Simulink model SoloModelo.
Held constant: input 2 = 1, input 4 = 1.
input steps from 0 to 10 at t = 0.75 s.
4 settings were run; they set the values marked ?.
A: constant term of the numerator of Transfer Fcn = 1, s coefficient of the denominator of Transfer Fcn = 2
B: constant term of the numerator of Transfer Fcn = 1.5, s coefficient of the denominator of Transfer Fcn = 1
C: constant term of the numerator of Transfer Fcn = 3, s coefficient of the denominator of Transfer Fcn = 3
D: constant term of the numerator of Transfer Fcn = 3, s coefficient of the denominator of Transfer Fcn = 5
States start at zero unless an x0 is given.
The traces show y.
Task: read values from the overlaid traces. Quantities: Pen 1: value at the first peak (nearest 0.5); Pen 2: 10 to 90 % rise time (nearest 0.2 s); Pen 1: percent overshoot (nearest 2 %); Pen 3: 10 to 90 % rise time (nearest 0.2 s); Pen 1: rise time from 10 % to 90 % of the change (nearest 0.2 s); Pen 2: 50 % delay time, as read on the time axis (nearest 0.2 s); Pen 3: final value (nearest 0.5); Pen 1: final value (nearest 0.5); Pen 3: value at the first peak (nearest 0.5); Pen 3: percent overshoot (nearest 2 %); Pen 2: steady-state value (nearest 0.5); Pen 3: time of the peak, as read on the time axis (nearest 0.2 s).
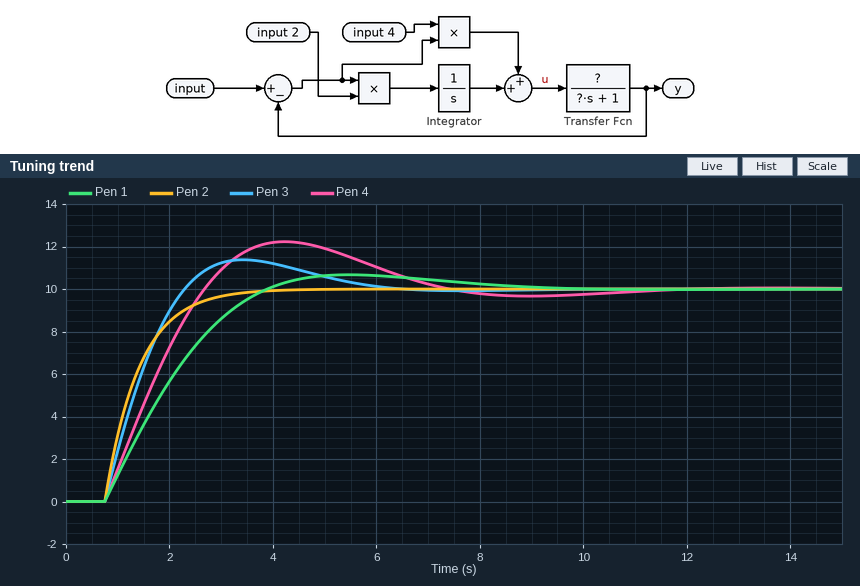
10.5
1.4 s
6 %
1.2 s
2.2 s
1.2 s
10.0
10.0
11.5
14 %
10.0
3.4 s
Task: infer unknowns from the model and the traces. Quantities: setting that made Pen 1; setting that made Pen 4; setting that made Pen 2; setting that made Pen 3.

A
D
B
C
